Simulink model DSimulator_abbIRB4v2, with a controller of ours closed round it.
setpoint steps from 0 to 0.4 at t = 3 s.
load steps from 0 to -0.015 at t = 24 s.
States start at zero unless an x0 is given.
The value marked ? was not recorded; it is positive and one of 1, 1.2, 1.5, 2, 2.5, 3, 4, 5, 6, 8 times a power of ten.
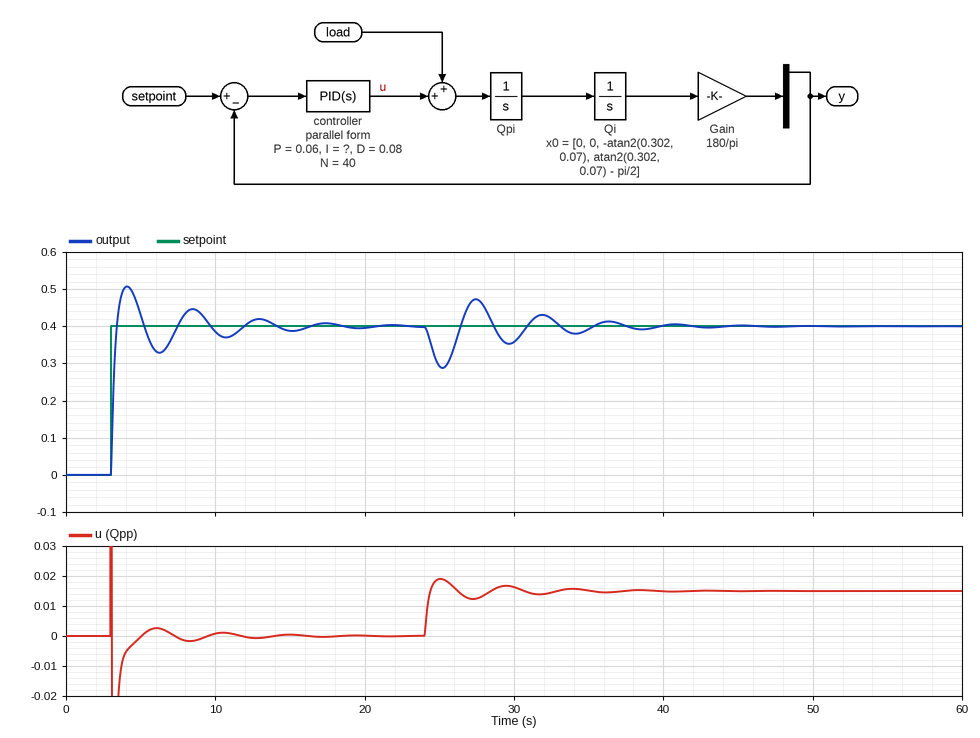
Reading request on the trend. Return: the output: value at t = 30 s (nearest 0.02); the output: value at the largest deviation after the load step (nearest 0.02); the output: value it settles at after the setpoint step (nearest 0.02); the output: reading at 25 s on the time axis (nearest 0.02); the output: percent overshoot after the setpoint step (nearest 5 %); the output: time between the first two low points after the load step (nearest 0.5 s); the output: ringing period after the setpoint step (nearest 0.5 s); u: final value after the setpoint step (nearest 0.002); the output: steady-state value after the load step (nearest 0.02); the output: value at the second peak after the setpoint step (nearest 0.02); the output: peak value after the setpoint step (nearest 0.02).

0.36
0.28
0.40
0.30
25 %
4.5 s
4.5 s
0.000
0.40
0.44
0.50
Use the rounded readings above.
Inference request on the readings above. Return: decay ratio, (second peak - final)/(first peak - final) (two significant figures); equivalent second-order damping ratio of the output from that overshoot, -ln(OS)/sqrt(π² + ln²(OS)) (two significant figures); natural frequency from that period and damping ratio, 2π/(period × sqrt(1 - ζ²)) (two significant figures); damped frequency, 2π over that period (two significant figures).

0.40
0.40
1.5 rad/s
1.4 rad/s
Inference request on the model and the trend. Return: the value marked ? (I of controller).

0.15
